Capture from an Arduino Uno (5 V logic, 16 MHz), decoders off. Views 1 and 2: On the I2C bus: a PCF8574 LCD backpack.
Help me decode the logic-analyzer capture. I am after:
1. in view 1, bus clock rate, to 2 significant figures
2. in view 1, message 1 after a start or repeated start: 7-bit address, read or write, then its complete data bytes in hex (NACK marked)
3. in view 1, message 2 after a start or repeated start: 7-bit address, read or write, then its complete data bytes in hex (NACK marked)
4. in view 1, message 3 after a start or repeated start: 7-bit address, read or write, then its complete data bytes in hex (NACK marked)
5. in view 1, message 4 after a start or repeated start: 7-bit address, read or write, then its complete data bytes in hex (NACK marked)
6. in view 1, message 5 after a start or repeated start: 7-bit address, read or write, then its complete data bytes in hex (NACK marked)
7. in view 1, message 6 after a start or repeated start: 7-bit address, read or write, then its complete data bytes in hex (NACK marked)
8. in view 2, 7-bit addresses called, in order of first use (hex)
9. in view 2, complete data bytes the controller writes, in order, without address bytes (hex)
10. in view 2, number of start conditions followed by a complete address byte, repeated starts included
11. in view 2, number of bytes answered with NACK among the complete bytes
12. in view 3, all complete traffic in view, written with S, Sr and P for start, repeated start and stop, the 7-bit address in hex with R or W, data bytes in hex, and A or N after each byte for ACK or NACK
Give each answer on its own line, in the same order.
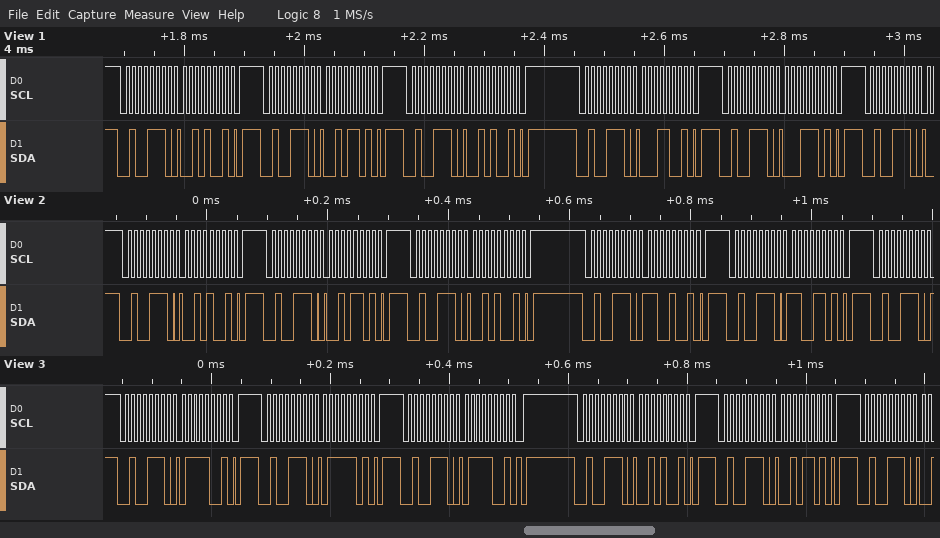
100 kHz
0x27 write: 29
0x27 write: 2D
0x27 write: 29
0x27 write: 19
0x27 write: 1D
0x27 write
0x27
29 2D 29 C9 CD
6
0
S 27W A 79 A P S 27W A 7D A P S 27W A 79 A P S 27W A 29 A P S 27W A 2D A P S 27W A
